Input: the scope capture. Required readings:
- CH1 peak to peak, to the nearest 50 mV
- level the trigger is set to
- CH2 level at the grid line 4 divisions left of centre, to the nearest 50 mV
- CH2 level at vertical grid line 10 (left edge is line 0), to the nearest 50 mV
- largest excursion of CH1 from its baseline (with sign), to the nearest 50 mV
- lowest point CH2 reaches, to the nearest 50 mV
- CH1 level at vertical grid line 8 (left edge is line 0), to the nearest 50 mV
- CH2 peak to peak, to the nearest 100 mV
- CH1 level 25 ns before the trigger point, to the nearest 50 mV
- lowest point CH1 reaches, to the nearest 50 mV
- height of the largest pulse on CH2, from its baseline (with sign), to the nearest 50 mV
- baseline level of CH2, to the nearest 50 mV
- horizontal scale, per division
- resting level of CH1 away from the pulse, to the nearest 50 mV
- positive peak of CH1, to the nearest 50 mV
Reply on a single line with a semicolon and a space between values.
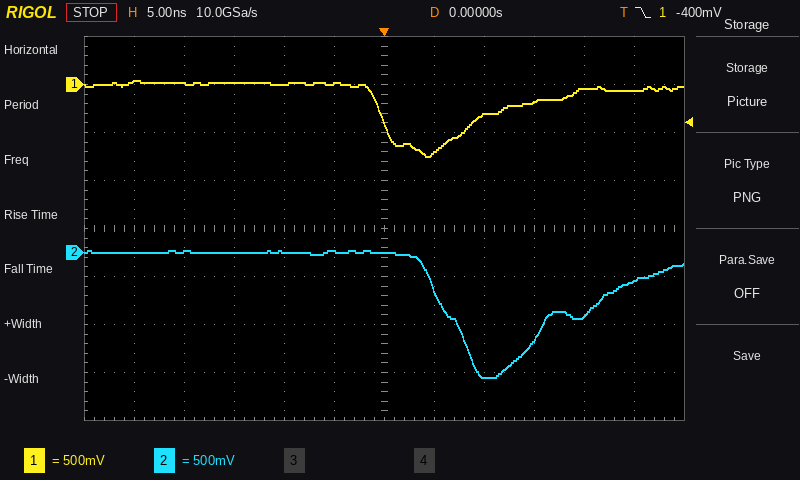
800 mV; -400 mV; 0 mV; -650 mV; -750 mV; -1.30 V; -300 mV; 1.30 V; 50 mV; -750 mV; -1.30 V; 0 mV; 5 ns; 0 mV; 50 mV
